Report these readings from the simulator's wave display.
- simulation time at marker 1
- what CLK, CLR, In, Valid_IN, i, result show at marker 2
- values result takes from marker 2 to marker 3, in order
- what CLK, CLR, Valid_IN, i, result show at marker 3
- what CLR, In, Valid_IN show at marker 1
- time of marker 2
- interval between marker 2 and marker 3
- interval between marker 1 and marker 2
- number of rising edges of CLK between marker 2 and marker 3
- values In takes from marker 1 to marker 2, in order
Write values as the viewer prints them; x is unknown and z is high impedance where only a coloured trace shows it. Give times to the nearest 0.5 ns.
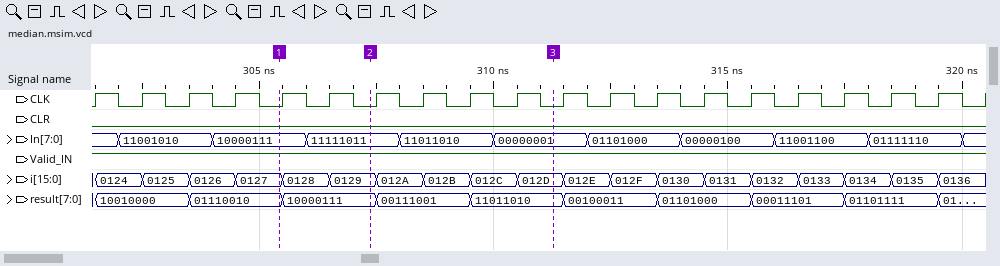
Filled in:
305.5 ns
CLK=0, CLR=0, In=11111011, Valid_IN=1, i=0129, result=10000111
10000111, 00111001, 11011010
CLK=0, CLR=0, Valid_IN=1, i=012D, result=11011010
CLR=0, In=10000111, Valid_IN=1
307.5 ns
4 ns
2 ns
4
10000111, 11111011
